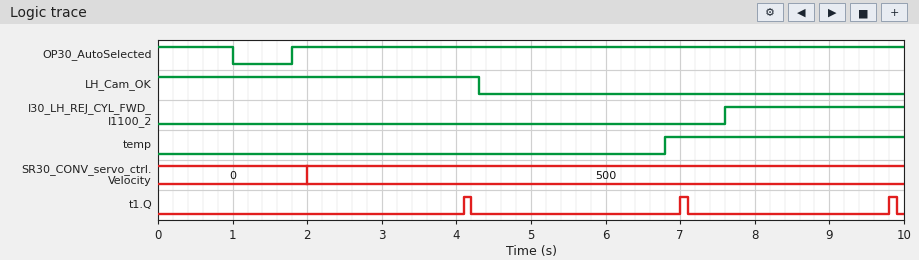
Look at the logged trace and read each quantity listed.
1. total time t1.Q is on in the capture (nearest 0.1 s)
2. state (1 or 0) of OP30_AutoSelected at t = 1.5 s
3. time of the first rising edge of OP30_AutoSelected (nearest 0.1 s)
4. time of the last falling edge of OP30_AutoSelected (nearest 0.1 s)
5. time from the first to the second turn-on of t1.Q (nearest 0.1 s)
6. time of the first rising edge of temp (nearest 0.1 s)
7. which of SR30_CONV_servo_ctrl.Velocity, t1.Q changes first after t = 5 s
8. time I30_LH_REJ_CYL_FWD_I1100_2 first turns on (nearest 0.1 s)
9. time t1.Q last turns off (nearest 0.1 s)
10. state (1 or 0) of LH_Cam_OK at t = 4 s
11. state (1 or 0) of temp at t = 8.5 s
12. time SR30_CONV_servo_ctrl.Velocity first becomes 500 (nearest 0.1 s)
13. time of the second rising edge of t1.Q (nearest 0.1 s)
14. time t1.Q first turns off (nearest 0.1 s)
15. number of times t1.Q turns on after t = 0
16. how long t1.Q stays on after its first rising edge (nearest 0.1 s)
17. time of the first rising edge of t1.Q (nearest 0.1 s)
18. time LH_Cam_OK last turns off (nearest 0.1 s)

0.3 s
0
1.8 s
1.0 s
2.9 s
6.8 s
t1.Q
7.6 s
9.9 s
1
1
2.0 s
7.0 s
4.2 s
3
0.1 s
4.1 s
4.3 s
